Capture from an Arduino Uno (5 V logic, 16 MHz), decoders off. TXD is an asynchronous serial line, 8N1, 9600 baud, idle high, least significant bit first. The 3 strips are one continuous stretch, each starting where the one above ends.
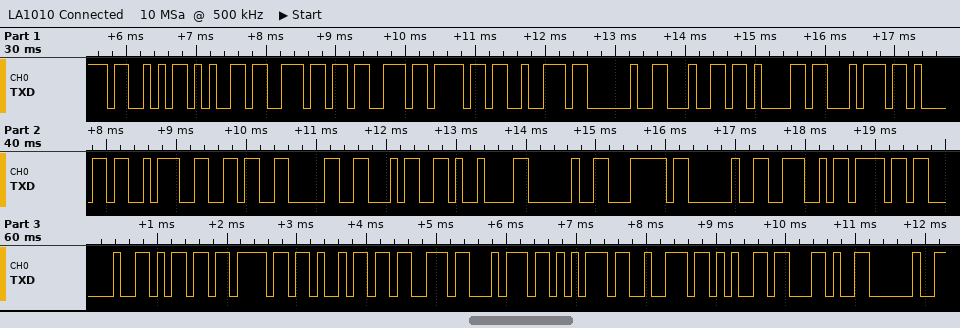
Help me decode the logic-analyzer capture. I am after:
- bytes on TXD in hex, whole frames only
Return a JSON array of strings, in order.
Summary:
["53 65 6E 73 6F 72 20 64 61 74 61 3A 36 30 34 09 20 7C 20 4E 6F 20 6D 6F 69 73 74 75 72 65 2C 20"]
